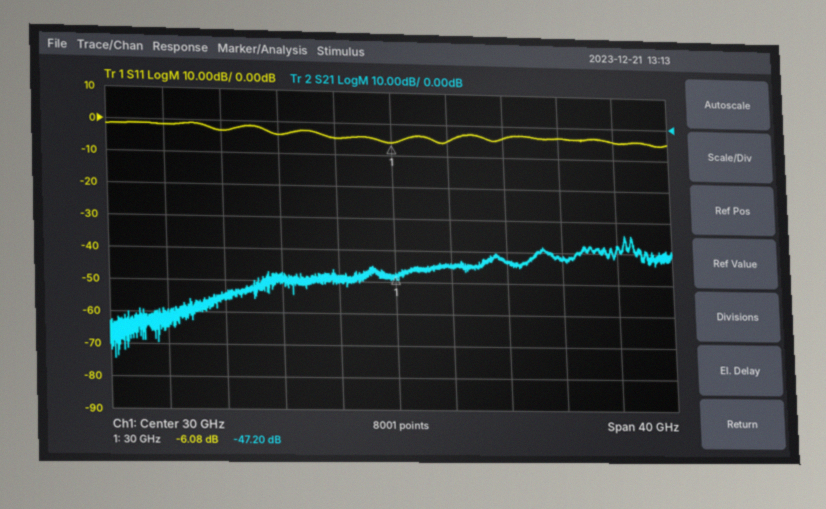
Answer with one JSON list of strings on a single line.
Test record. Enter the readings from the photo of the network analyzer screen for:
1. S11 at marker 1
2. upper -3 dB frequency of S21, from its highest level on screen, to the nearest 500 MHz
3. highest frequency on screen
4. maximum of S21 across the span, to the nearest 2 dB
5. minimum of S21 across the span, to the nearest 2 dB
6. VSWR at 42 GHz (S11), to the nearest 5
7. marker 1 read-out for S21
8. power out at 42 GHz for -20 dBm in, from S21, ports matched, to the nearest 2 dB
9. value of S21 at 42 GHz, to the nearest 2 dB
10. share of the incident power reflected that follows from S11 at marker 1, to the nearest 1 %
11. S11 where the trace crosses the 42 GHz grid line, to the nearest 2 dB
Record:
["-6.08 dB", "46.5 GHz", "50 GHz", "-34 dB", "-74 dB", "5", "-47.20 dB", "-62 dBm", "-42 dB", "25 %", "-4 dB"]
